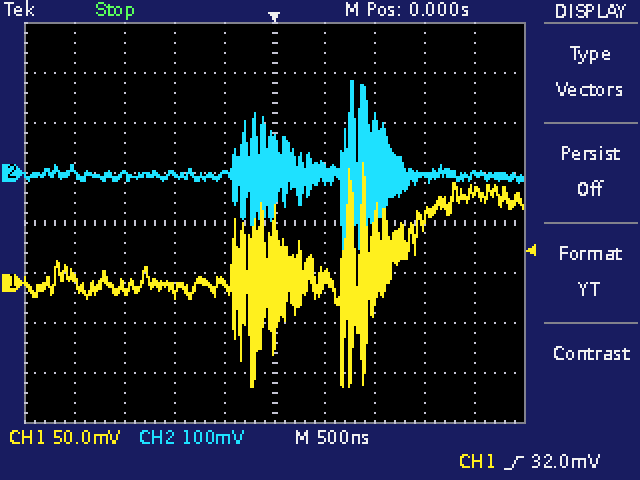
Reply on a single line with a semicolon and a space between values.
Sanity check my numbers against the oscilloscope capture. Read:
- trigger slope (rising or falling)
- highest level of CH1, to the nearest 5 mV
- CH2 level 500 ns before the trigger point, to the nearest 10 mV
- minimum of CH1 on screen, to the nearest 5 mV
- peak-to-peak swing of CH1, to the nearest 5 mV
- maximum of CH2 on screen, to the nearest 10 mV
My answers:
rising; 120 mV; 0 mV; -105 mV; 225 mV; 180 mV
